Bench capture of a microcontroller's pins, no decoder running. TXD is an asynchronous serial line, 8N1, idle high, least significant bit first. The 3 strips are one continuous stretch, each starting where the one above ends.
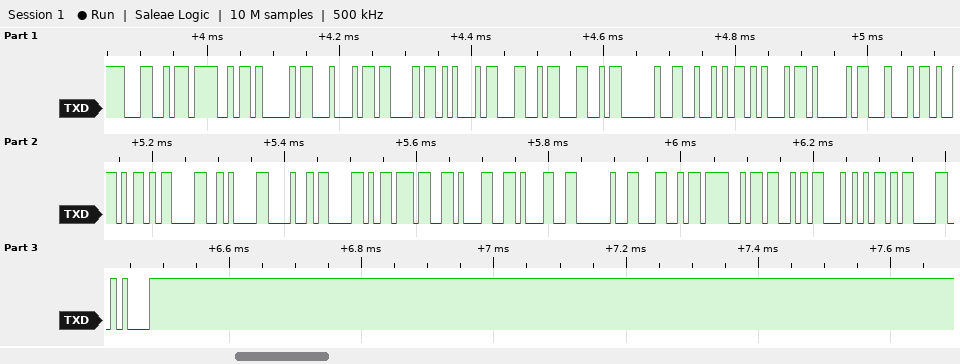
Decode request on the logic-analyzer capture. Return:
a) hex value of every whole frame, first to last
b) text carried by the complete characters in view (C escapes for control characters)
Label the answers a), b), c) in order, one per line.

a) 4C 4F 41 44 43 45 4C 4C 20 52 45 41 44 59 0D 0A 48 58 37 31 31 20 4C 4F 53 54 0D 0A
b) "LOADCELL READY\r\nHX711 LOST\r\n"
